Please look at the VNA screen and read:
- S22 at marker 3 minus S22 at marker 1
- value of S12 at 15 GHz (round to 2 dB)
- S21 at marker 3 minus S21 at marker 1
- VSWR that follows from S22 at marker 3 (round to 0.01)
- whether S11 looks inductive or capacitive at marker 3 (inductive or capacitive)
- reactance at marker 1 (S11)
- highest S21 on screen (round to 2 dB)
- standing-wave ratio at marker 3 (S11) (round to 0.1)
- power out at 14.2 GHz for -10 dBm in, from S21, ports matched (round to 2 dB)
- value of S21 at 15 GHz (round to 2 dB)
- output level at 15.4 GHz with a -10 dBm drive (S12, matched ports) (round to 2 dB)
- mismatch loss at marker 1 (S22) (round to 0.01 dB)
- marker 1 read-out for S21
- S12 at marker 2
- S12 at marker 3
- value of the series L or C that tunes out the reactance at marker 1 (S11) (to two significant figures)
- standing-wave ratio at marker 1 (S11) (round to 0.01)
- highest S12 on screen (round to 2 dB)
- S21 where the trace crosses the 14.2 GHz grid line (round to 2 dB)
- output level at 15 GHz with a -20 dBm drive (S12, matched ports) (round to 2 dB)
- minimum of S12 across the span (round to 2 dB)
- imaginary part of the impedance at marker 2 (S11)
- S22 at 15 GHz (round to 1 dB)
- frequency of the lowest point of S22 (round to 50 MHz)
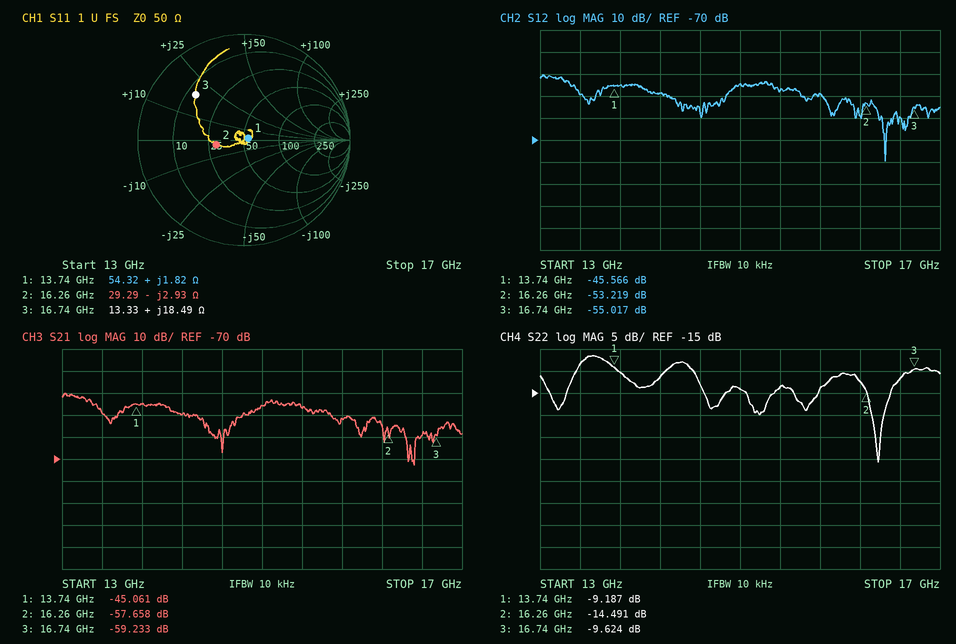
-0.437 dB
-44 dB
-14.172 dB
1.99
inductive
+1.82 Ω
-40 dB
4.3
-60 dBm
-46 dB
-58 dBm
0.56 dB
-45.061 dB
-53.219 dB
-55.017 dB
6.4 pF
1.09
-40 dB
-50 dB
-64 dBm
-80 dB
-2.93 Ω
-14 dB
16.40 GHz
